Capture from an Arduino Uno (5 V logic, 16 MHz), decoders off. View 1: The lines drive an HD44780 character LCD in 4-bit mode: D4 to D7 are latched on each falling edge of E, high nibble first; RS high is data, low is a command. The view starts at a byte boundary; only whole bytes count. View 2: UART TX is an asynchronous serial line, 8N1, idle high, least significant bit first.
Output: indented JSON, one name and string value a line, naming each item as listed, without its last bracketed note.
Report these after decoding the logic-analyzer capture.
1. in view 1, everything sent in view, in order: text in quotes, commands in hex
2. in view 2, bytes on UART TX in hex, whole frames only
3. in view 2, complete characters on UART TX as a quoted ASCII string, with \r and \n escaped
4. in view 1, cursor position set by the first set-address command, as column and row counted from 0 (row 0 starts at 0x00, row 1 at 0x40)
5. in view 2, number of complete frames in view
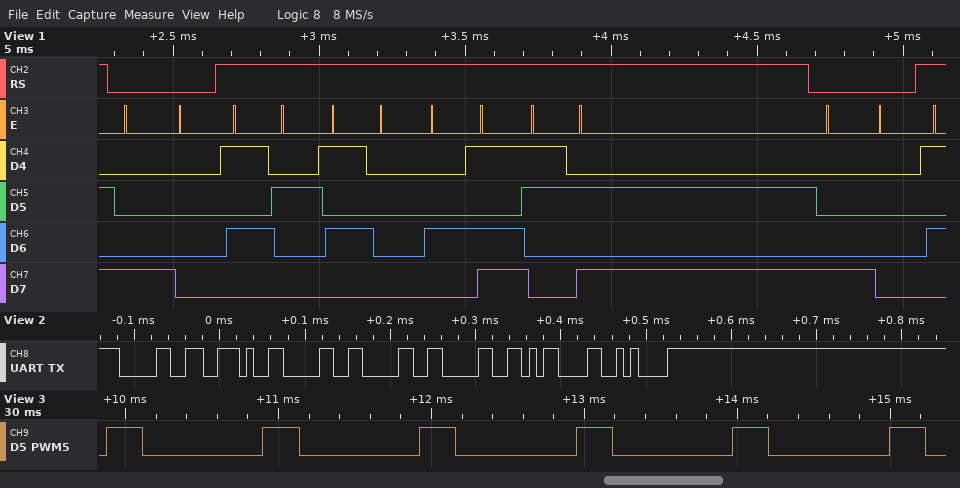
{
  "in view 1, everything sent in view, in order: text in quotes, commands in hex": "0x80 \"RPM:\" 0x80",
  "in view 2, bytes on UART TX in hex, whole frames only": "30 2E 30 30 30 0D 0A",
  "in view 2, complete characters on UART TX as a quoted ASCII string, with \\r and \\n escaped": "\"0.000\\r\\n\"",
  "in view 1, cursor position set by the first set-address command, as column and row counted from 0": "column 0, row 0",
  "in view 2, number of complete frames in view": "7"
}
